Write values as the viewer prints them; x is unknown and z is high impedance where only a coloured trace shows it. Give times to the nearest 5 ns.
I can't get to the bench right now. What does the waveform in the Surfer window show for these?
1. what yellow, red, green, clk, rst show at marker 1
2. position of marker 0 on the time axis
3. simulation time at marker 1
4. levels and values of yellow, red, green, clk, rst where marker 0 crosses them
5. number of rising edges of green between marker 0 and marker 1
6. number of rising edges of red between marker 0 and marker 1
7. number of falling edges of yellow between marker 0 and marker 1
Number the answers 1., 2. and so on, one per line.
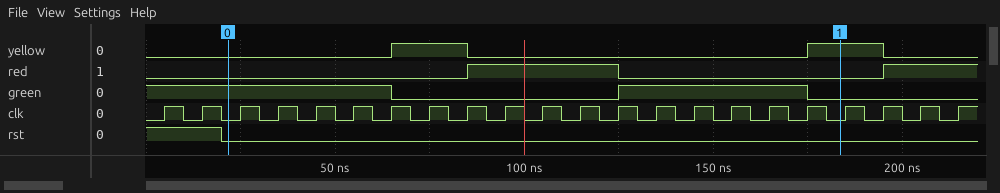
1. yellow=1, red=0, green=0, clk=0, rst=0
2. 20 ns
3. 185 ns
4. yellow=0, red=0, green=1, clk=0, rst=0
5. 1
6. 1
7. 1
